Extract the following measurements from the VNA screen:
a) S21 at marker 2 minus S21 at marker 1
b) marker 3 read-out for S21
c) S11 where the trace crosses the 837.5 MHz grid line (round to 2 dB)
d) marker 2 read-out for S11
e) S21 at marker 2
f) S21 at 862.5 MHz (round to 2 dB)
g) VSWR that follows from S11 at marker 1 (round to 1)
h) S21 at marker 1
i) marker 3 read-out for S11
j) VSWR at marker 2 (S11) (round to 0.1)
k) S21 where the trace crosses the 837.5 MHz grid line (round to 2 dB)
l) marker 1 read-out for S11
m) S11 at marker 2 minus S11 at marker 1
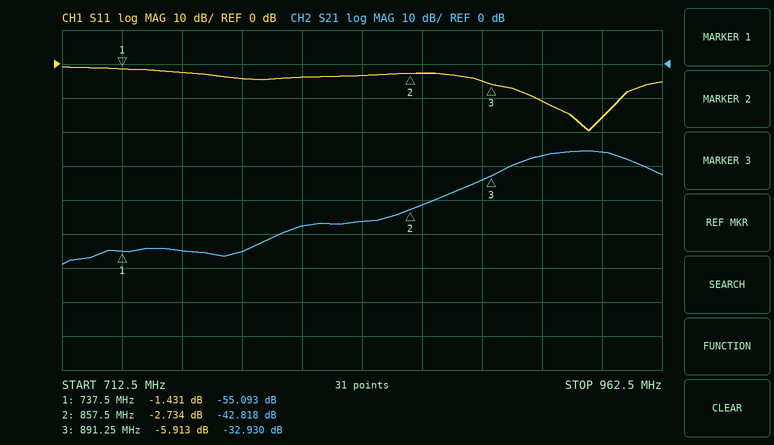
12.275 dB
-32.930 dB
-4 dB
-2.734 dB
-42.818 dB
-42 dB
12
-55.093 dB
-5.913 dB
6.4
-46 dB
-1.431 dB
-1.303 dB
